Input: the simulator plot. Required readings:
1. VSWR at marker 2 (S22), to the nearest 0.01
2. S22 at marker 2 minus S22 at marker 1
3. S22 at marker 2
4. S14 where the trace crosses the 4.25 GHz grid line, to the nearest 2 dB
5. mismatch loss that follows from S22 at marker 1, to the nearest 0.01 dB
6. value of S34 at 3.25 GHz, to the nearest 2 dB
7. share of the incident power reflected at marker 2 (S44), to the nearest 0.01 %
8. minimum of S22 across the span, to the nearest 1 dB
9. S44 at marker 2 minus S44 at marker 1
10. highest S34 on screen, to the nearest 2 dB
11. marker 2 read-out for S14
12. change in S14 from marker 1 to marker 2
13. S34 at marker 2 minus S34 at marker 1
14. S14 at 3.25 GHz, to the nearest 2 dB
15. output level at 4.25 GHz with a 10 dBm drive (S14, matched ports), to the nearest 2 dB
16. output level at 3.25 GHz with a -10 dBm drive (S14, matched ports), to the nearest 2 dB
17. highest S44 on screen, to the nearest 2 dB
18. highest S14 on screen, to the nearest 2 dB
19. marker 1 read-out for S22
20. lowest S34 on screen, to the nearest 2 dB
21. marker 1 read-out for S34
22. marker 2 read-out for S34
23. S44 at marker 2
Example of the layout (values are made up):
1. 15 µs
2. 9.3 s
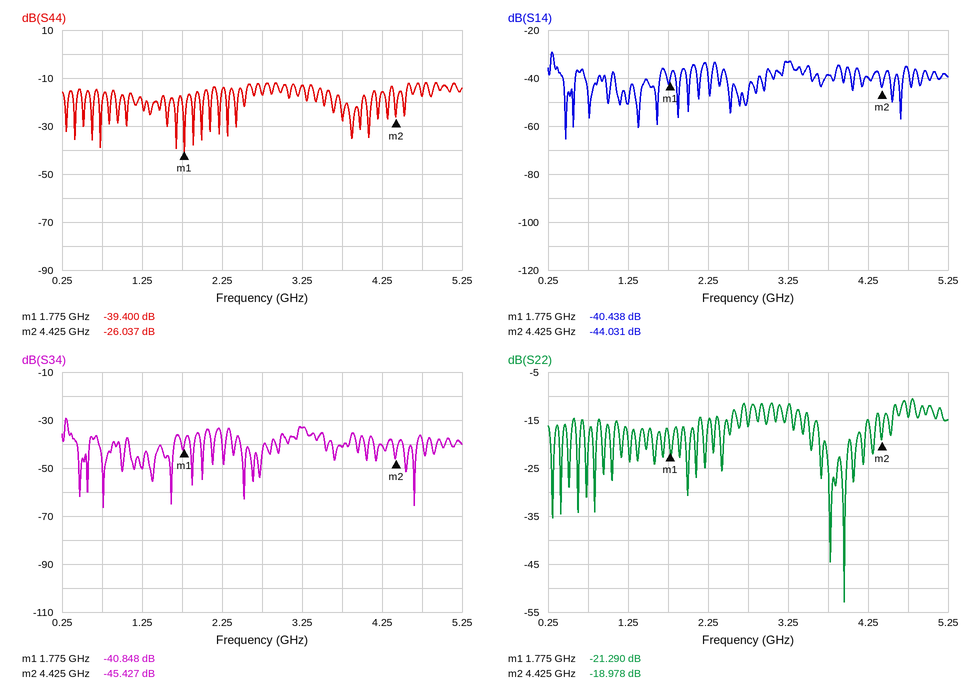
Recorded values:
1. 1.25
2. 2.312 dB
3. -18.978 dB
4. -40 dB
5. 0.03 dB
6. -34 dB
7. 0.25 %
8. -53 dB
9. 13.363 dB
10. -30 dB
11. -44.031 dB
12. -3.593 dB
13. -4.579 dB
14. -34 dB
15. -30 dBm
16. -44 dBm
17. -12 dB
18. -30 dB
19. -21.290 dB
20. -66 dB
21. -40.848 dB
22. -45.427 dB
23. -26.037 dB
